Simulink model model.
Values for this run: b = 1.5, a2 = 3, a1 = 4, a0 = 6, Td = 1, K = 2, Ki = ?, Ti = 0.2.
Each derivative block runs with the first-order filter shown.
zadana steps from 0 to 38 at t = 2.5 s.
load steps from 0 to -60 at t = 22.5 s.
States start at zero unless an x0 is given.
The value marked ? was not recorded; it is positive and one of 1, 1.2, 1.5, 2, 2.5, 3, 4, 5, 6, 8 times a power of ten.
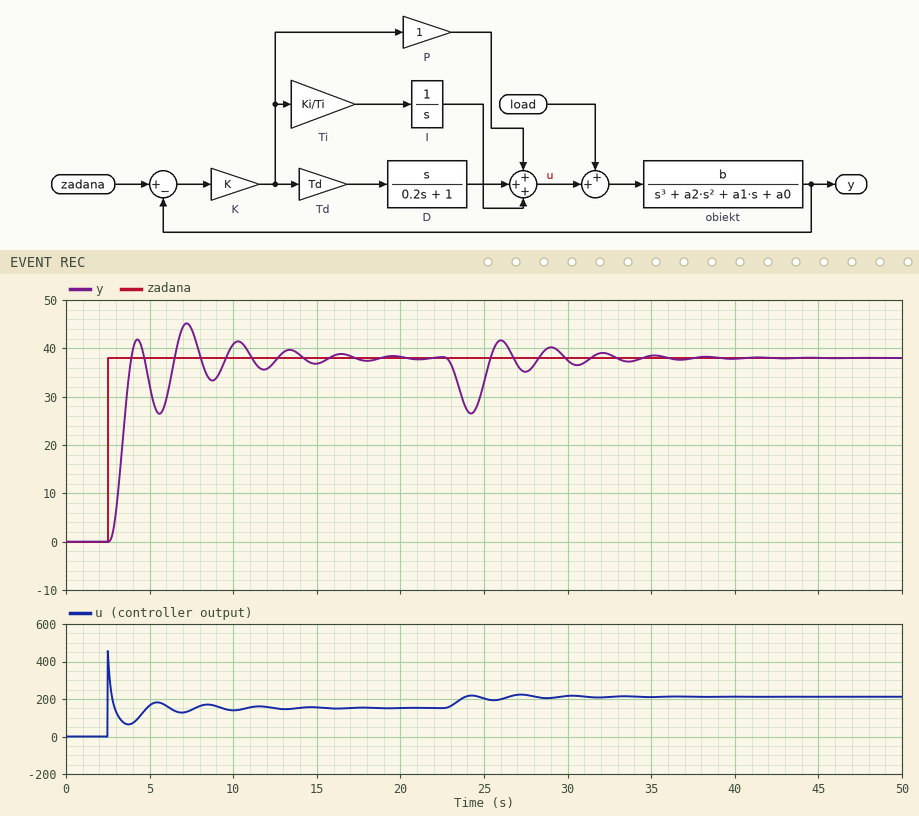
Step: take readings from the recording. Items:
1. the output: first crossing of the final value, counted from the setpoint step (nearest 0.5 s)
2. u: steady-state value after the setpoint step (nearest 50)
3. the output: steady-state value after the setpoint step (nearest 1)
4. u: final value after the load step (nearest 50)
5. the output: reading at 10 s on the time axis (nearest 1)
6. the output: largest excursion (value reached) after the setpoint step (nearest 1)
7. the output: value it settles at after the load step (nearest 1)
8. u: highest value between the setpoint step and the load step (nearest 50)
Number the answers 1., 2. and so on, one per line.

1. 1.5 s
2. 150
3. 38
4. 200
5. 41
6. 45
7. 38
8. 450
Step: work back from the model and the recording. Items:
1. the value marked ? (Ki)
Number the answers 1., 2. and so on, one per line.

1. 0.4
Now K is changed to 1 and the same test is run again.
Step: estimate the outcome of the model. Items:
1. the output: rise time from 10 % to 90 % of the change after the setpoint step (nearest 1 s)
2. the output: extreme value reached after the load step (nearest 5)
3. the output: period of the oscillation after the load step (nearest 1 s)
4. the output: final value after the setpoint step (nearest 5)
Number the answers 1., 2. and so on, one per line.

1. 4 s
2. 25
3. 4 s
4. 40
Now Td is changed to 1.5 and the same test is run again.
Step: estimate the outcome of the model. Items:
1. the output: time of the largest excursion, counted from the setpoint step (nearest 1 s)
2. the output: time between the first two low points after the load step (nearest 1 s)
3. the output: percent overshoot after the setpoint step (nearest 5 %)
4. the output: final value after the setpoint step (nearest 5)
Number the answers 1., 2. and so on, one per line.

1. 4 s
2. 3 s
3. 15 %
4. 40
